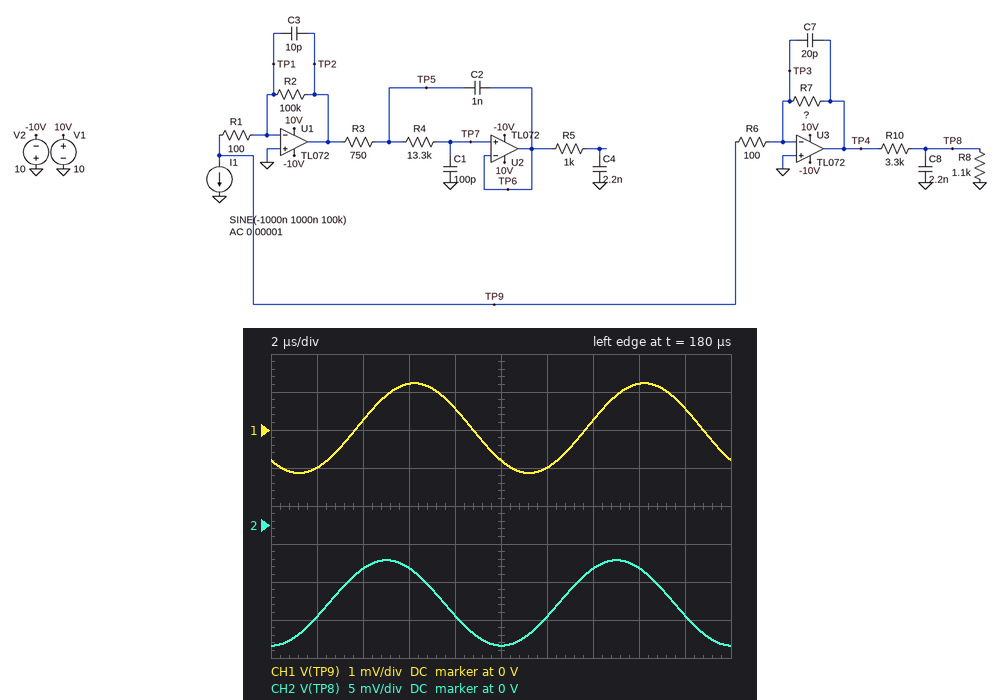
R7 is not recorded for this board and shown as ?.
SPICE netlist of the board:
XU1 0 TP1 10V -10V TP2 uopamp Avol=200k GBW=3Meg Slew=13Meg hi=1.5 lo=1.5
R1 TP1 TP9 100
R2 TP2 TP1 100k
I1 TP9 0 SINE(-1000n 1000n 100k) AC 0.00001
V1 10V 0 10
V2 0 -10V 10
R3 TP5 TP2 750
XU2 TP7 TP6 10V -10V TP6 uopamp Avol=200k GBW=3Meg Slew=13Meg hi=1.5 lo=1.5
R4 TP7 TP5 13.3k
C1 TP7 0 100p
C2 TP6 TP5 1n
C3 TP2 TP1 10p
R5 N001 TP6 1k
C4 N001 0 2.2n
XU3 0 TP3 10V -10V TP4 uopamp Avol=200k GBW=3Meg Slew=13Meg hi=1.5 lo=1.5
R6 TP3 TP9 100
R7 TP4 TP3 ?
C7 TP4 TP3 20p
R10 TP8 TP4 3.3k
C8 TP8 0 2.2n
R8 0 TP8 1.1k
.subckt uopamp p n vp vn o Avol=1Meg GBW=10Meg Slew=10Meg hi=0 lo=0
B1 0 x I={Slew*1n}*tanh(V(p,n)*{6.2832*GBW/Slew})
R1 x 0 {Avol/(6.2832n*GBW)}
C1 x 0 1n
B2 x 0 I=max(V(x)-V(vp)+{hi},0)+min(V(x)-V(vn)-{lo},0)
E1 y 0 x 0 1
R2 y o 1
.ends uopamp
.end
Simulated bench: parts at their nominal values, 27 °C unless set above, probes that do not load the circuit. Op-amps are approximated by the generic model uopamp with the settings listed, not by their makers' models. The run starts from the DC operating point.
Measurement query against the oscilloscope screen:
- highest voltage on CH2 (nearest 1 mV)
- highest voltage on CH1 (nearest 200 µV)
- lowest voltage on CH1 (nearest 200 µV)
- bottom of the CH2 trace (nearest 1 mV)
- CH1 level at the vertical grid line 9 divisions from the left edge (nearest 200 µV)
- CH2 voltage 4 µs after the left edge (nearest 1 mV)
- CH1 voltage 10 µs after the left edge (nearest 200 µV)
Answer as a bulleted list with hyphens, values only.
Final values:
- -5 mV
- 1.2 mV
- -1.2 mV
- -16 mV
- 600 µV
- -6 mV
- -800 µV
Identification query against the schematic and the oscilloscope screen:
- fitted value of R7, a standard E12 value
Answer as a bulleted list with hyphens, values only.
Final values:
- 82 kΩ
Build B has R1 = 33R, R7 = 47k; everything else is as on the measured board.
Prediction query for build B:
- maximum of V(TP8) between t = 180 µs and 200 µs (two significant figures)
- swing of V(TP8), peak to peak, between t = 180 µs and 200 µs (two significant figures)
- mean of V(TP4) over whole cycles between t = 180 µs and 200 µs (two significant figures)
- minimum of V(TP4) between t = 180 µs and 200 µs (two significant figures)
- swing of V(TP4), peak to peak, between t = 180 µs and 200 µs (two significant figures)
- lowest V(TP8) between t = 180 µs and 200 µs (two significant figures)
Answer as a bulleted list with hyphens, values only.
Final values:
- 1.5 mV
- 8.9 mV
- -12 mV
- -39 mV
- 54 mV
- -7.4 mV
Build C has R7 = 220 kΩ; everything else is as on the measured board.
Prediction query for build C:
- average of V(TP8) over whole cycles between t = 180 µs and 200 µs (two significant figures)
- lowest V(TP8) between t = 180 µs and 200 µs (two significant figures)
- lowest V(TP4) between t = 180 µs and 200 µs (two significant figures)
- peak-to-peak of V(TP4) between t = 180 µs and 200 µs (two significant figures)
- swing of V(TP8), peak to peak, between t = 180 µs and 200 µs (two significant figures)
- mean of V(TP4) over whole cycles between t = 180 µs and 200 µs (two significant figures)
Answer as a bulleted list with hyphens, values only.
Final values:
- -27 mV
- -34 mV
- -150 mV
- 83 mV
- 14 mV
- -110 mV
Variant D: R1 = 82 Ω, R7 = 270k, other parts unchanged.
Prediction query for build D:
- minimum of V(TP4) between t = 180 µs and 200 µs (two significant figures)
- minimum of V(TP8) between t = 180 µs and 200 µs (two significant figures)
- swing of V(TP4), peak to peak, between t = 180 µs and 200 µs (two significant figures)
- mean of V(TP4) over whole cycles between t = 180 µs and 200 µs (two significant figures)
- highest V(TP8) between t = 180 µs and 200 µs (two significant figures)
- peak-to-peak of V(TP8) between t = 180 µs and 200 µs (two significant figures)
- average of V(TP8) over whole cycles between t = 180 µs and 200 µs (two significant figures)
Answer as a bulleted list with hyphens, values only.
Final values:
- -160 mV
- -37 mV
- 85 mV
- -120 mV
- -23 mV
- 14 mV
- -30 mV
